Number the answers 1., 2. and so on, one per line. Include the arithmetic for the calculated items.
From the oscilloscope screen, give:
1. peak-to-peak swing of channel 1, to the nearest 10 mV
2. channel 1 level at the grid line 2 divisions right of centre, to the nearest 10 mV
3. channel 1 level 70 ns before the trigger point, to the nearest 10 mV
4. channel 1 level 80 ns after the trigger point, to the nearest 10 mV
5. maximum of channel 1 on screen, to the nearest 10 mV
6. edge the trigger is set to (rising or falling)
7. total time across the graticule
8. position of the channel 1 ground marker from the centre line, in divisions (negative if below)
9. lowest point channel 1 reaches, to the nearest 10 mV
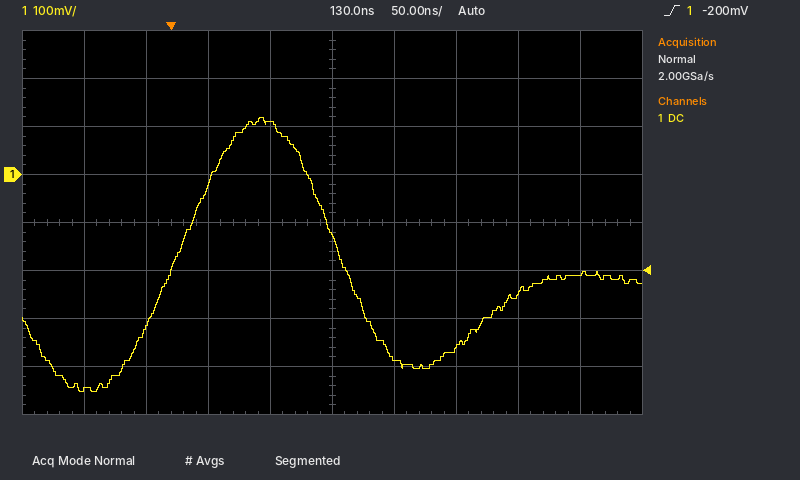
1. 120 mV − (-450 mV) = 570 mV
2. -360 mV
3. -450 mV
4. 110 mV
5. 120 mV
6. rising
7. 500 ns
8. +1.0 div
9. -450 mV
